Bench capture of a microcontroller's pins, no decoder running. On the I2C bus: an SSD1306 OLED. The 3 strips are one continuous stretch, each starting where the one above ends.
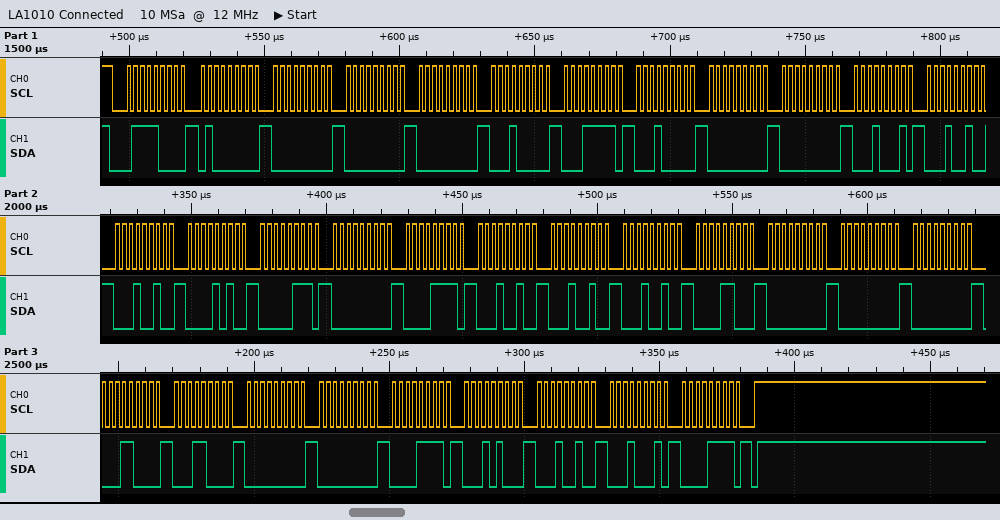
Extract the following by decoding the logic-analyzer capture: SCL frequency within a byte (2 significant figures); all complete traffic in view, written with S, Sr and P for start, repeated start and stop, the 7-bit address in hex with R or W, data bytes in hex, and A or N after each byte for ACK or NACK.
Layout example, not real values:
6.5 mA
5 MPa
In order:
400 kHz
S 3CW A 40 A 00 A 00 A 00 A 10 A 1F A 10 A 00 A 00 A 11 A 12 A 12 A 0A A 07 A 00 A 0F A 12 A 12 A 12 A 0C A 00 A 00 A 00 A 18 A 18 A 00 A 00 A 0F A 14 A 12 A 11 A 0F A P
